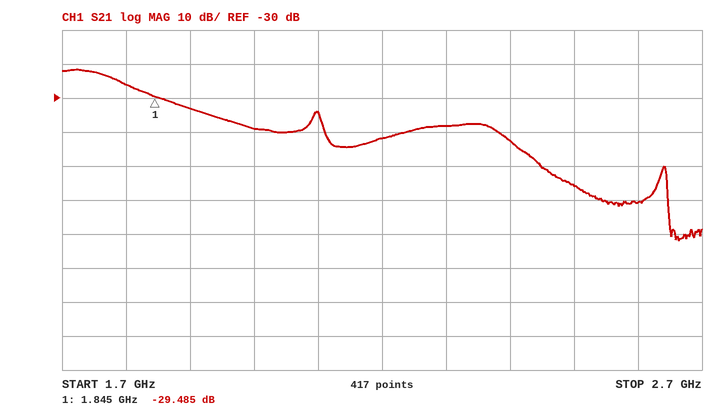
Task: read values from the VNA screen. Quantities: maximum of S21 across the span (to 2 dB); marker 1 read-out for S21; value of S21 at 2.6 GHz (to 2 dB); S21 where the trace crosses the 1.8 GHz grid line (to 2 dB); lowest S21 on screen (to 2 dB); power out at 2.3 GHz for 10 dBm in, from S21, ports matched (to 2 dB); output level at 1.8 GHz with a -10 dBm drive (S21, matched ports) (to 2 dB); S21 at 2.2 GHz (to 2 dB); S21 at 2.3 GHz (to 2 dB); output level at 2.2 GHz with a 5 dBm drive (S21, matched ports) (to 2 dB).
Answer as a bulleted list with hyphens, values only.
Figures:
- -22 dB
- -29.485 dB
- -60 dB
- -26 dB
- -72 dB
- -28 dBm
- -36 dBm
- -42 dB
- -38 dB
- -36 dBm
